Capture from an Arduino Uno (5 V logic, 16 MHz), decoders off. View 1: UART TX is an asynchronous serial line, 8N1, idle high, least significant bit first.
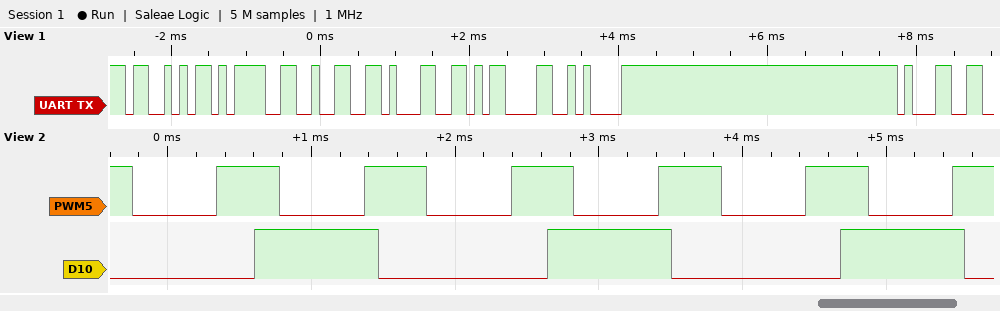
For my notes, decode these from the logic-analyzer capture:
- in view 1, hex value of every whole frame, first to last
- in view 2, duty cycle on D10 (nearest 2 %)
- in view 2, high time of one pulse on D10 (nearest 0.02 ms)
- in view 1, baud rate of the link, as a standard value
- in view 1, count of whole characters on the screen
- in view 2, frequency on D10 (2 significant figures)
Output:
53 3D 32 31 0D 0A 31
42 %
0.86 ms
9600 baud
7
490 Hz
